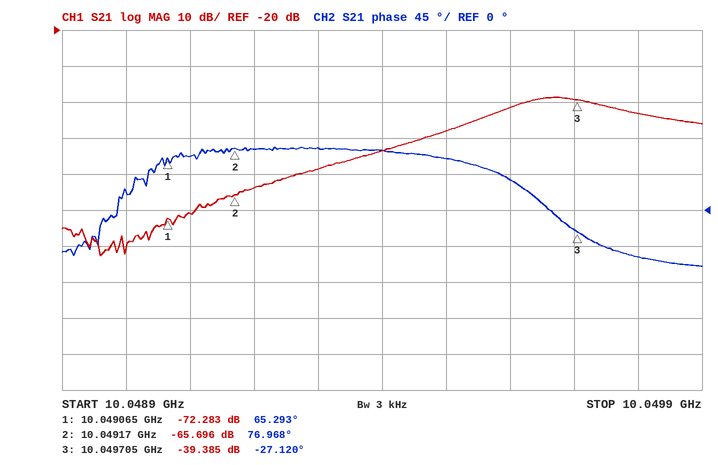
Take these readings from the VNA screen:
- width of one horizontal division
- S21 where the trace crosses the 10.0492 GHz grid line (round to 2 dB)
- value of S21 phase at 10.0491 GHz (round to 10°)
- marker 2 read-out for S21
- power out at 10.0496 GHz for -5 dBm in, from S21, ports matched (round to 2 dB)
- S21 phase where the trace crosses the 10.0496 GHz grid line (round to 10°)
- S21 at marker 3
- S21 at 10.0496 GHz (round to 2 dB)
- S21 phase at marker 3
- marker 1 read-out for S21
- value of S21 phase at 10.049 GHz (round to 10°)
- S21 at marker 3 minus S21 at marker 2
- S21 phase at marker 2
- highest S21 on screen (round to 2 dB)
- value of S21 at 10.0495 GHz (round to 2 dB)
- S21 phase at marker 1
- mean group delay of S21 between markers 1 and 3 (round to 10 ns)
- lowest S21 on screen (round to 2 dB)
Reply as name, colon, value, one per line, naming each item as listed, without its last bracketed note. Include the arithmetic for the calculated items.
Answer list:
width of one horizontal division: 100 kHz
S21 where the trace crosses the 10.0492 GHz grid line: -64 dB
value of S21 phase at 10.0491 GHz: 70°
marker 2 read-out for S21: -65.696 dB
power out at 10.0496 GHz for -5 dBm in, from S21, ports matched: -5 dBm + (-42 dB) = -46 dBm
S21 phase where the trace crosses the 10.0496 GHz grid line: 40°
S21 at marker 3: -39.385 dB
S21 at 10.0496 GHz: -42 dB
S21 phase at marker 3: -27.120°
marker 1 read-out for S21: -72.283 dB
value of S21 phase at 10.049 GHz: 20°
S21 at marker 3 minus S21 at marker 2: -39.385 − (-65.696) = 26.311 dB
S21 phase at marker 2: 76.968°
highest S21 on screen: -38 dB
value of S21 at 10.0495 GHz: -48 dB
S21 phase at marker 1: 65.293°
mean group delay of S21 between markers 1 and 3: −(-27.12° − (65.293°))/(360° × 640 kHz) ≈ 401 ns, so 400 ns to the nearest 10 ns
lowest S21 on screen: -82 dB
